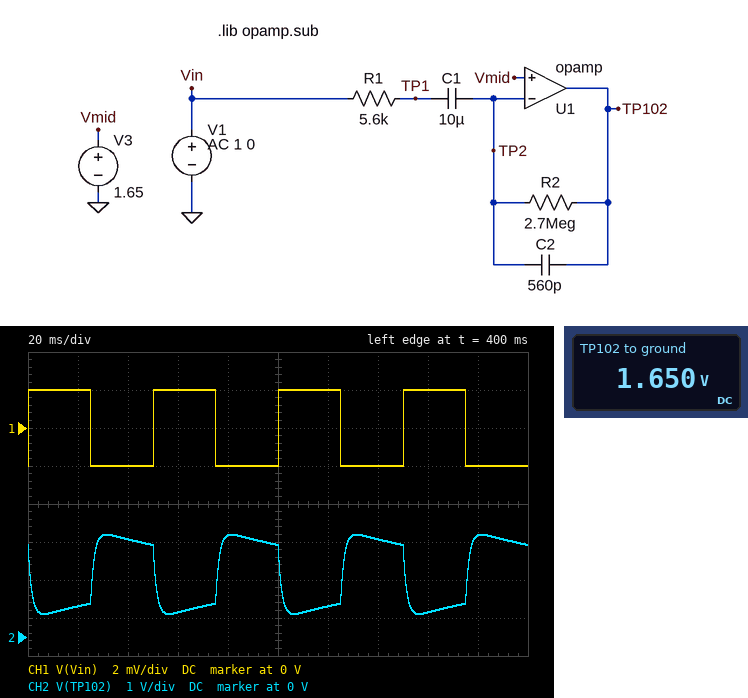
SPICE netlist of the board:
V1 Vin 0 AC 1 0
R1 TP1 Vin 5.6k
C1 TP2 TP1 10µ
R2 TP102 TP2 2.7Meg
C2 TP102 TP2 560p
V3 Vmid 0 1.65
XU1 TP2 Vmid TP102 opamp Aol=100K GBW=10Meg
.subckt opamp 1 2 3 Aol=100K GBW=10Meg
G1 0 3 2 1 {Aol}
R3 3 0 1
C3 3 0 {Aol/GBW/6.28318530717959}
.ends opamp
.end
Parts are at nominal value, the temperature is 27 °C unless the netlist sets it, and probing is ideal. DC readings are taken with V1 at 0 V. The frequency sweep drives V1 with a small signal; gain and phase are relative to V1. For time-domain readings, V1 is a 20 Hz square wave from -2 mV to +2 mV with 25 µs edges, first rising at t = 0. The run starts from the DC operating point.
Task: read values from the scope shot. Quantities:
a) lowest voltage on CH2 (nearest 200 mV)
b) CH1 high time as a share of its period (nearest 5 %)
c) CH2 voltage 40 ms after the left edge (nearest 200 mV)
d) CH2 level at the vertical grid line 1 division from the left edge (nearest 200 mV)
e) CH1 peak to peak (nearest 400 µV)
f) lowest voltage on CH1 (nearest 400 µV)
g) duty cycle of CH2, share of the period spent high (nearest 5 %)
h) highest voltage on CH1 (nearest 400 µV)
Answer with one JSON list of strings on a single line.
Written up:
["600 mV", "50 %", "2.6 V", "800 mV", "4.0 mV", "-2.0 mV", "50 %", "2.0 mV"]
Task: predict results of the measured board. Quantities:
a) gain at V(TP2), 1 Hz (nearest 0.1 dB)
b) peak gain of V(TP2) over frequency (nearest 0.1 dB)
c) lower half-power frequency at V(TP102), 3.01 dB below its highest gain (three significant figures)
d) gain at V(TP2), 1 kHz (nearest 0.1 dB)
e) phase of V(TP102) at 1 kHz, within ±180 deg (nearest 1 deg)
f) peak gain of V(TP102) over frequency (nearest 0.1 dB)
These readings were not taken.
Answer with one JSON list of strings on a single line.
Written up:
["-55.9 dB", "-45.9 dB", "2.69 Hz", "-45.9 dB", "96 deg", "53.4 dB"]
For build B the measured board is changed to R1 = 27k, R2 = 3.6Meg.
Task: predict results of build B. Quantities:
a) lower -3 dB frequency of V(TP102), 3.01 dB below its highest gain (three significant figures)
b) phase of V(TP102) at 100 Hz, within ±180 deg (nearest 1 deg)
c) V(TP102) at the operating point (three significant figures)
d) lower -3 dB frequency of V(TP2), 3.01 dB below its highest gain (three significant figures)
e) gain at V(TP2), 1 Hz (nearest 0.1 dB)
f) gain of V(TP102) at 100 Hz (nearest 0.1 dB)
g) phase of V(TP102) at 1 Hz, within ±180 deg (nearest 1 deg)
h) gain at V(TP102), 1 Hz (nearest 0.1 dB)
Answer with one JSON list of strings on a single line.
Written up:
["580 mHz", "129 deg", "1.65 V", "583 mHz", "-58.8 dB", "38.3 dB", "-150 deg", "41.2 dB"]
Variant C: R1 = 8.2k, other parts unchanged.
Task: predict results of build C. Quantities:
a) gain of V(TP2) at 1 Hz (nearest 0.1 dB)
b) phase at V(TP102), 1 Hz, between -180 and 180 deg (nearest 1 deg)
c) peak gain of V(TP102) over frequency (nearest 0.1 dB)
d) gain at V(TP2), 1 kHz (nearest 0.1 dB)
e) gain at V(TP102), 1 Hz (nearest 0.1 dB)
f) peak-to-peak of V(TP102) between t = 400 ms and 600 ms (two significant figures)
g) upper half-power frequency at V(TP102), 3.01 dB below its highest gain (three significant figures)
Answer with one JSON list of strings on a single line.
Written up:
["-56.4 dB", "-118 deg", "50.2 dB", "-49.2 dB", "43.6 dB", "1.4 V", "109 Hz"]
